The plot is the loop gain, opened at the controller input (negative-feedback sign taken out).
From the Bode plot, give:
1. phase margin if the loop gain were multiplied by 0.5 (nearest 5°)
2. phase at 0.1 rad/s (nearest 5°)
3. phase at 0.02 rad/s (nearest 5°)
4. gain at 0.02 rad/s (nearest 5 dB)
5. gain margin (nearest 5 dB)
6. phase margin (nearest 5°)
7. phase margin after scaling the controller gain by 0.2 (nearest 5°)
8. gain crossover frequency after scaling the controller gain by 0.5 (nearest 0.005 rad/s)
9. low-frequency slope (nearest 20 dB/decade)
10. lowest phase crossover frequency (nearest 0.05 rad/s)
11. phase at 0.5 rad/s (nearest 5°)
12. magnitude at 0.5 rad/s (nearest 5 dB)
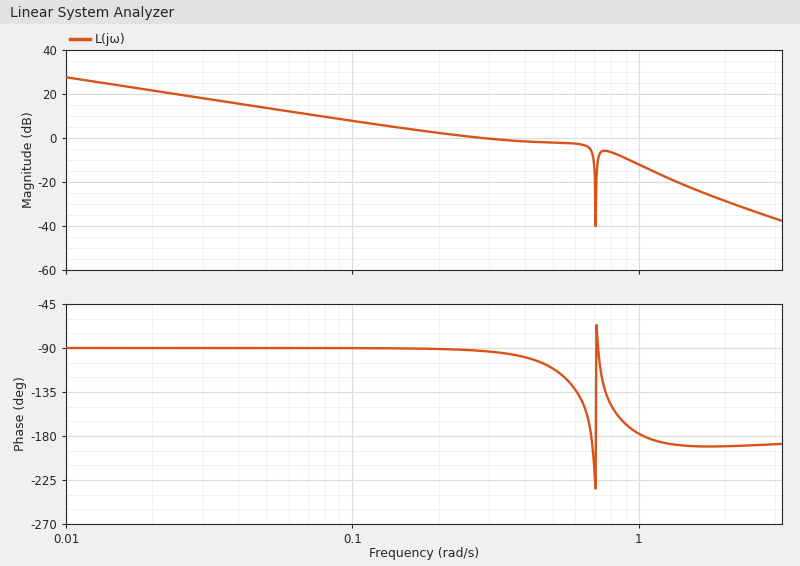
90°
-90°
-90°
20 dB
5 dB
85°
90°
0.125 rad/s
-20 dB/decade
0.70 rad/s
-110°
0 dB
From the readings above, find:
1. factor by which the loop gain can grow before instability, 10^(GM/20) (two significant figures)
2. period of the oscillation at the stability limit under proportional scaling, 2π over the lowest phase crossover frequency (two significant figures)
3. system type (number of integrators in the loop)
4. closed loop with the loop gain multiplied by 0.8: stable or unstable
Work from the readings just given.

1.8
9.0 s
1
stable
